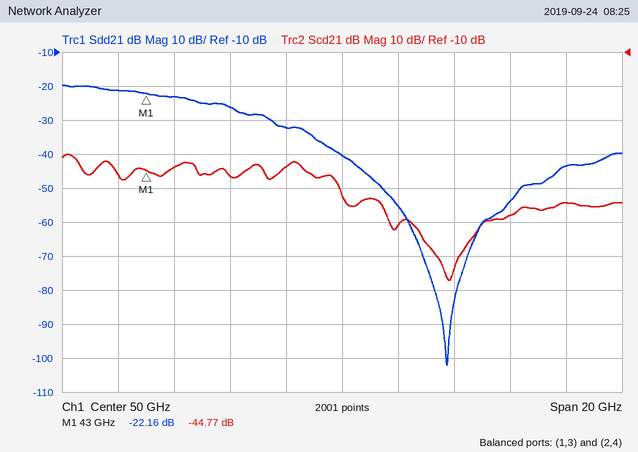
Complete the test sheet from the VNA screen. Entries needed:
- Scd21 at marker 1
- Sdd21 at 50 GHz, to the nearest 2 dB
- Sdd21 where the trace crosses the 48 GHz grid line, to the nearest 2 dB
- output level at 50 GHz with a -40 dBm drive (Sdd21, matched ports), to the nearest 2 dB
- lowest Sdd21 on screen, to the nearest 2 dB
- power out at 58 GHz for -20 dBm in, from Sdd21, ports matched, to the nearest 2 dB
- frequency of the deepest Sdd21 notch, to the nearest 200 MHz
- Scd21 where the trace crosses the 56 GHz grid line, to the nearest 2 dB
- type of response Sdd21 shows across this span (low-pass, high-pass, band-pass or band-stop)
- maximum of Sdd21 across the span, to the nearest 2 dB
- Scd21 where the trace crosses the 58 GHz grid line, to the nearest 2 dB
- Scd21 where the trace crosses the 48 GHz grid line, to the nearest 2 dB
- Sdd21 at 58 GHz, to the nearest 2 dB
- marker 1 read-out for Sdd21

-44.77 dB
-40 dB
-32 dB
-80 dBm
-102 dB
-64 dBm
53.8 GHz
-58 dB
low-pass
-20 dB
-54 dB
-44 dB
-44 dB
-22.16 dB
